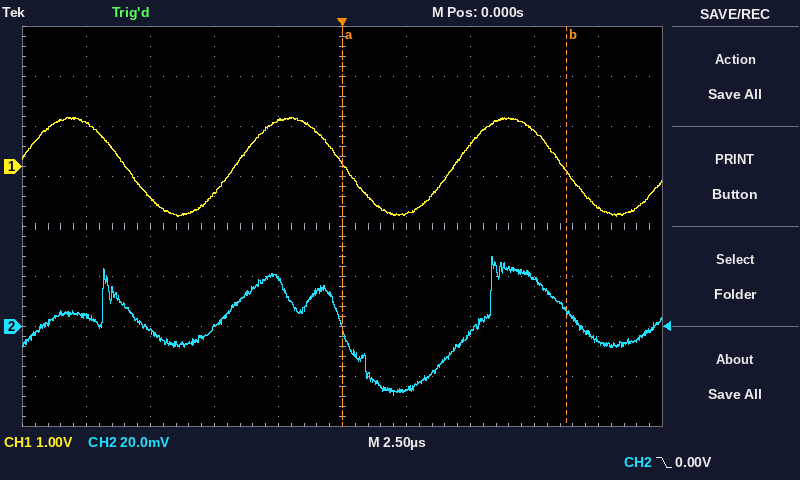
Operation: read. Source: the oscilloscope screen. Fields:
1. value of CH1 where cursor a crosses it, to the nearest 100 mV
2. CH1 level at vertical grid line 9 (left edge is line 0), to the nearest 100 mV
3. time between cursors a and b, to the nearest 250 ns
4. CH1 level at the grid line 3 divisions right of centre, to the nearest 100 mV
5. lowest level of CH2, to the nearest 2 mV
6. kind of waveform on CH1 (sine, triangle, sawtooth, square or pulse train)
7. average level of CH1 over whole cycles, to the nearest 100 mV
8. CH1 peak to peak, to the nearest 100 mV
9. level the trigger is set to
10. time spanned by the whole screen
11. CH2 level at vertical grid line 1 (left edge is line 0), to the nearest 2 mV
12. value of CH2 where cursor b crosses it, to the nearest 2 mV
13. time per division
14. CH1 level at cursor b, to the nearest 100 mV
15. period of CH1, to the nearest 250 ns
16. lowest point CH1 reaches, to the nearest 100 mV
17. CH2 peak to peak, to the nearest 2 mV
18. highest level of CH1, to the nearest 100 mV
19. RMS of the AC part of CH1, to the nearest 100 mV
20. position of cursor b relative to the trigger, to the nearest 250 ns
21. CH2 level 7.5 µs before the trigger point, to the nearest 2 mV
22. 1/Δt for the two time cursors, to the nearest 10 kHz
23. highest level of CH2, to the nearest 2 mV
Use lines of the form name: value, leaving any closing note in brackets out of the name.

value of CH1 where cursor a crosses it, to the nearest 100 mV: 100 mV
CH1 level at vertical grid line 9 (left edge is line 0), to the nearest 100 mV: -800 mV
time between cursors a and b, to the nearest 250 ns: 8.75 µs
CH1 level at the grid line 3 divisions right of centre, to the nearest 100 mV: 700 mV
lowest level of CH2, to the nearest 2 mV: -28 mV
kind of waveform on CH1: sine
average level of CH1 over whole cycles, to the nearest 100 mV: 0.0 V
CH1 peak to peak, to the nearest 100 mV: 2.0 V
level the trigger is set to: 0.00 V
time spanned by the whole screen: 25 µs
CH2 level at vertical grid line 1 (left edge is line 0), to the nearest 2 mV: 4 mV
value of CH2 where cursor b crosses it, to the nearest 2 mV: 6 mV
time per division: 2.5 µs
CH1 level at cursor b, to the nearest 100 mV: -100 mV
period of CH1, to the nearest 250 ns: 8.50 µs
lowest point CH1 reaches, to the nearest 100 mV: -1.0 V
CH2 peak to peak, to the nearest 2 mV: 56 mV
highest level of CH1, to the nearest 100 mV: 1.0 V
RMS of the AC part of CH1, to the nearest 100 mV: 700 mV
position of cursor b relative to the trigger, to the nearest 250 ns: +8.75 µs
CH2 level 7.5 µs before the trigger point, to the nearest 2 mV: -2 mV
1/Δt for the two time cursors, to the nearest 10 kHz: 110 kHz
highest level of CH2, to the nearest 2 mV: 28 mV
